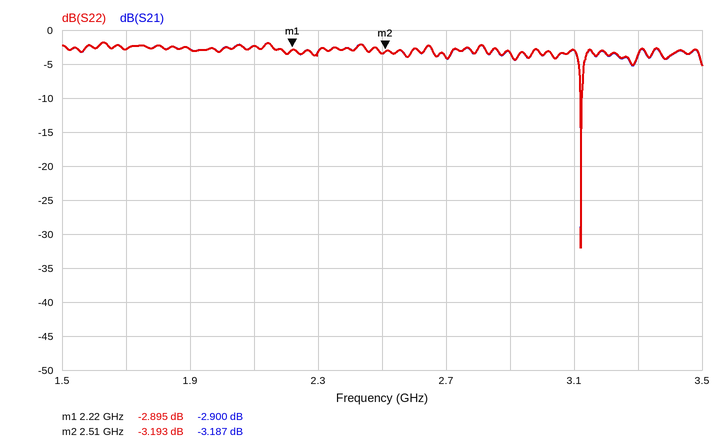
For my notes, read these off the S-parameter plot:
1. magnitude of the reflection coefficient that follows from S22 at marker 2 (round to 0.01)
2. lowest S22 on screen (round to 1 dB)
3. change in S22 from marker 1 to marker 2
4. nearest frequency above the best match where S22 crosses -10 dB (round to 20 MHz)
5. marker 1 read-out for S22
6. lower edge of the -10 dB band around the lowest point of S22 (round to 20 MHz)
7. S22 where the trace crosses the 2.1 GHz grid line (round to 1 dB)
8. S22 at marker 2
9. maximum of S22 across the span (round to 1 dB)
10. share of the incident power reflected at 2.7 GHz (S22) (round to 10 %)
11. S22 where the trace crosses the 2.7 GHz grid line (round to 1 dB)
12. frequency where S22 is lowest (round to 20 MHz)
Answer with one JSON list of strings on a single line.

["0.69", "-32 dB", "-0.298 dB", "3.12 GHz", "-2.895 dB", "3.12 GHz", "-2 dB", "-3.193 dB", "-2 dB", "40 %", "-4 dB", "3.12 GHz"]
